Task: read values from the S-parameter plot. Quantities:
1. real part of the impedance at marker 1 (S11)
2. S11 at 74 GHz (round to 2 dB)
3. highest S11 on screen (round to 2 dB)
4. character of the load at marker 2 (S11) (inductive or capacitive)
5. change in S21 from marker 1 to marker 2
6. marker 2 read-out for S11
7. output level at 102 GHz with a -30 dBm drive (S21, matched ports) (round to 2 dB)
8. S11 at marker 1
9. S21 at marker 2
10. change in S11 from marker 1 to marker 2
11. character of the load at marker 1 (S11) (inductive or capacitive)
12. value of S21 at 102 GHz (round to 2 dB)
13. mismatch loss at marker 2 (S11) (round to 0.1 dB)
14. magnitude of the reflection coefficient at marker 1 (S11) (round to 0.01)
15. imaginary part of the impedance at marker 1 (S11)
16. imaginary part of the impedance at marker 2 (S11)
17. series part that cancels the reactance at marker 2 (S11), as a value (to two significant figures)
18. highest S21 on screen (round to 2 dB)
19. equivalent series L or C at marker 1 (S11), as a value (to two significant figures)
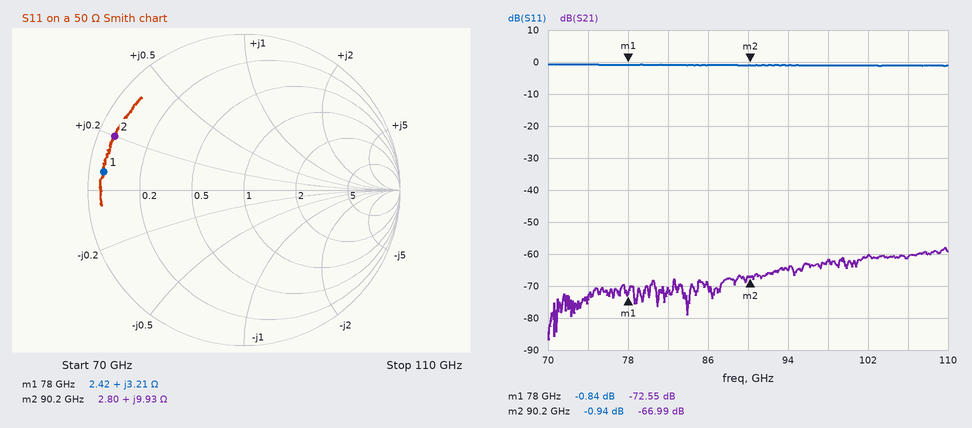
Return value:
2.42 Ω
0 dB
0 dB
inductive
5.56 dB
-0.94 dB
-90 dBm
-0.84 dB
-66.99 dB
-0.10 dB
inductive
-60 dB
7.1 dB
0.91
+3.21 Ω
+9.93 Ω
180 fF
-58 dB
6.5 pH
